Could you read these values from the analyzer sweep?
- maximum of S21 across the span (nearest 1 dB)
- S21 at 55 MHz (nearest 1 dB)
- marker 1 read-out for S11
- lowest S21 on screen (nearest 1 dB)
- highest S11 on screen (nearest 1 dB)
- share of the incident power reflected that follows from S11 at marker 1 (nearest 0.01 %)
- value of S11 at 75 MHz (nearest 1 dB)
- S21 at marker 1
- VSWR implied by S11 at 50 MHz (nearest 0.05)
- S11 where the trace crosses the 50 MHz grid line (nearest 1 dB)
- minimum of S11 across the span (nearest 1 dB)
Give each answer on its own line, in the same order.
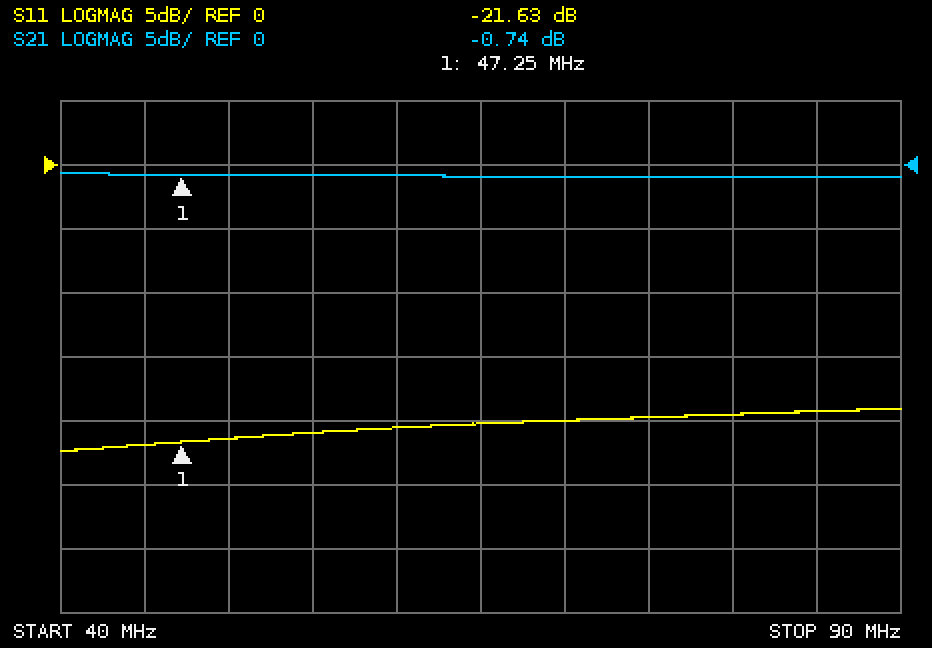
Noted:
-1 dB
-1 dB
-21.63 dB
-1 dB
-19 dB
0.69 %
-20 dB
-0.74 dB
1.20
-21 dB
-22 dB
